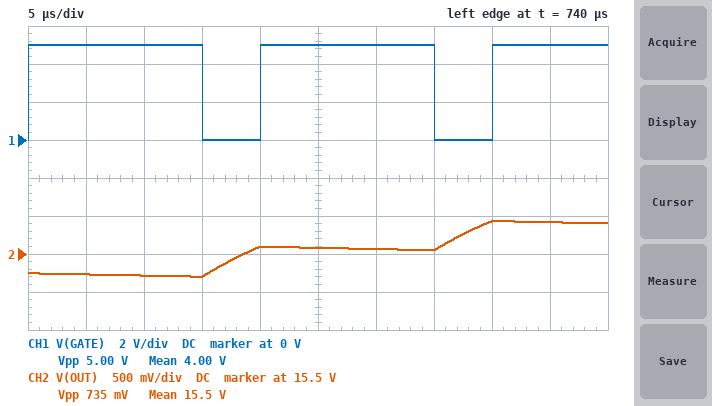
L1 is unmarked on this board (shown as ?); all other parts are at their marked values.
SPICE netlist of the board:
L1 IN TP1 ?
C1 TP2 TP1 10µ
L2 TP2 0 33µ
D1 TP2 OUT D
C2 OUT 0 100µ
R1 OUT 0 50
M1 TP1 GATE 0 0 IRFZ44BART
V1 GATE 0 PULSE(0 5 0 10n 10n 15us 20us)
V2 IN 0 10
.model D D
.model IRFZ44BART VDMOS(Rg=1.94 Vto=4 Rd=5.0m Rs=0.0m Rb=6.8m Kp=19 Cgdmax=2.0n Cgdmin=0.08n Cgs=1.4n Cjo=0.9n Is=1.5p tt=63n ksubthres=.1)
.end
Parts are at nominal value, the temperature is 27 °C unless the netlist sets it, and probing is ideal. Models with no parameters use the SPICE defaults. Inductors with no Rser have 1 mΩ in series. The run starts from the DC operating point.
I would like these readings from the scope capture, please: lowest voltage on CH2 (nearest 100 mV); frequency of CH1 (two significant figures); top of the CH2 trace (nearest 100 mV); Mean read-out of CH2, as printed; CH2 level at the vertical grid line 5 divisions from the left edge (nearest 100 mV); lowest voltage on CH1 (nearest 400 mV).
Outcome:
15.2 V
50 kHz
15.9 V
15.5 V
15.6 V
0 V
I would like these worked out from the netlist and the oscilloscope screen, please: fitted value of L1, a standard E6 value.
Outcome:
100 µH
